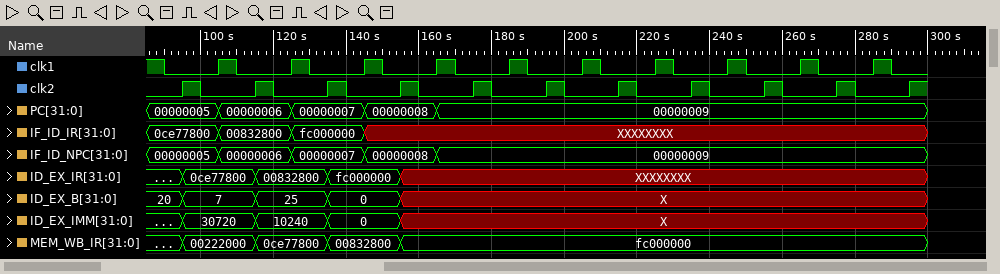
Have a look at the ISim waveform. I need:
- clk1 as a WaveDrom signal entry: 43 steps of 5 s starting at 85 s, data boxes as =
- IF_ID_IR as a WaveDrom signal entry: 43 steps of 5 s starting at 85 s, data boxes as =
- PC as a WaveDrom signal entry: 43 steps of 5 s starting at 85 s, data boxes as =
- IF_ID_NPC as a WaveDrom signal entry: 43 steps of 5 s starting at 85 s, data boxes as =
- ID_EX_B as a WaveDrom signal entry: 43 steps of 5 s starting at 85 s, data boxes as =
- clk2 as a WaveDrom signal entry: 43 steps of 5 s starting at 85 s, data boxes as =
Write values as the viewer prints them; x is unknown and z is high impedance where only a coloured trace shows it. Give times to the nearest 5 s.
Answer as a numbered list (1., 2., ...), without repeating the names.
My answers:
1. {name: 'clk1', wave: '10..10..10..10..10..10..10..10..10..10..10.'}
2. {name: 'IF_ID_IR', wave: '=...=...=...x..............................', data: '0ce77800 00832800 fc000000'}
3. {name: 'PC', wave: '=...=...=...=...=..........................', data: '00000005 00000006 00000007 00000008 00000009'}
4. {name: 'IF_ID_NPC', wave: '=...=...=...=...=..........................', data: '00000005 00000006 00000007 00000008 00000009'}
5. {name: 'ID_EX_B', wave: '=.=...=...=...x............................', data: '20 7 25 0'}
6. {name: 'clk2', wave: '0.10..10..10..10..10..10..10..10..10..10..1'}
